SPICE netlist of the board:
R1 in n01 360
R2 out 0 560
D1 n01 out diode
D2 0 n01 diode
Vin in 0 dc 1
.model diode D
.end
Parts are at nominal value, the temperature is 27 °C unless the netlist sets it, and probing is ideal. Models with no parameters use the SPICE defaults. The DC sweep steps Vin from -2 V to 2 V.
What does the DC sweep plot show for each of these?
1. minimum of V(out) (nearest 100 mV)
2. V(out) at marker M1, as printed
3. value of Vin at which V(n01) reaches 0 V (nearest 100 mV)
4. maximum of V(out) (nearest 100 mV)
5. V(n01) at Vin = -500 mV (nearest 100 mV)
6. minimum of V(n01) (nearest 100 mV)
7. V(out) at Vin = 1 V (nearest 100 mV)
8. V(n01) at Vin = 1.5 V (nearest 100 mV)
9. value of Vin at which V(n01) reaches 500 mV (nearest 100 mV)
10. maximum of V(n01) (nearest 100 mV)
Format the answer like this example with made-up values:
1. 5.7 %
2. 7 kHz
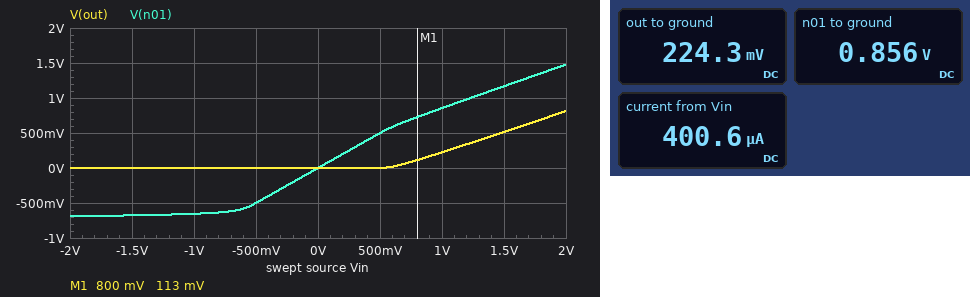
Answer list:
1. 0 V
2. 113 mV
3. 0 V
4. 800 mV
5. -500 mV
6. -700 mV
7. 200 mV
8. 1.2 V
9. 500 mV
10. 1.5 V
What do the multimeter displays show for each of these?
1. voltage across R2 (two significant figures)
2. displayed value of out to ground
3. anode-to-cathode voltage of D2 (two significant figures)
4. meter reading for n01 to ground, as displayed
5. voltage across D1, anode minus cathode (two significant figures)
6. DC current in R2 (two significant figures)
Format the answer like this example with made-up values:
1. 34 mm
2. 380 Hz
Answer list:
1. 220 mV
2. 224.3 mV
3. -860 mV
4. 0.856 V
5. 630 mV
6. 400 µA
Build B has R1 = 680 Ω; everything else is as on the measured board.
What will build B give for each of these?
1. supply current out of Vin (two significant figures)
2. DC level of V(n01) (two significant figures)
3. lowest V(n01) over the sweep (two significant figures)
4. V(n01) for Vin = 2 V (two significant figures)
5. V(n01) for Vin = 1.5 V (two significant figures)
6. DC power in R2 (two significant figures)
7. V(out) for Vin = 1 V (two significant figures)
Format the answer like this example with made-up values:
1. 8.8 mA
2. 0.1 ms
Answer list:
1. 300 µA
2. 790 mV
3. -670 mV
4. 1.3 V
5. 1.0 V
6. 51 µW
7. 170 mV
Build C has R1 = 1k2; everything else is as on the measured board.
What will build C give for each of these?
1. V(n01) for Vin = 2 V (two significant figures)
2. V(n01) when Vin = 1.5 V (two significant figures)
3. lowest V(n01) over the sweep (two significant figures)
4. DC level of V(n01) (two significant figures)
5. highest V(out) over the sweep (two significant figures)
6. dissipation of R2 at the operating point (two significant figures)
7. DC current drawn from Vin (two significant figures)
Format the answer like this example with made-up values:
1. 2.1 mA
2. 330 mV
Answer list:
1. 1.1 V
2. 910 mV
3. -660 mV
4. 740 mV
5. 430 mV
6. 27 µW
7. 220 µA
